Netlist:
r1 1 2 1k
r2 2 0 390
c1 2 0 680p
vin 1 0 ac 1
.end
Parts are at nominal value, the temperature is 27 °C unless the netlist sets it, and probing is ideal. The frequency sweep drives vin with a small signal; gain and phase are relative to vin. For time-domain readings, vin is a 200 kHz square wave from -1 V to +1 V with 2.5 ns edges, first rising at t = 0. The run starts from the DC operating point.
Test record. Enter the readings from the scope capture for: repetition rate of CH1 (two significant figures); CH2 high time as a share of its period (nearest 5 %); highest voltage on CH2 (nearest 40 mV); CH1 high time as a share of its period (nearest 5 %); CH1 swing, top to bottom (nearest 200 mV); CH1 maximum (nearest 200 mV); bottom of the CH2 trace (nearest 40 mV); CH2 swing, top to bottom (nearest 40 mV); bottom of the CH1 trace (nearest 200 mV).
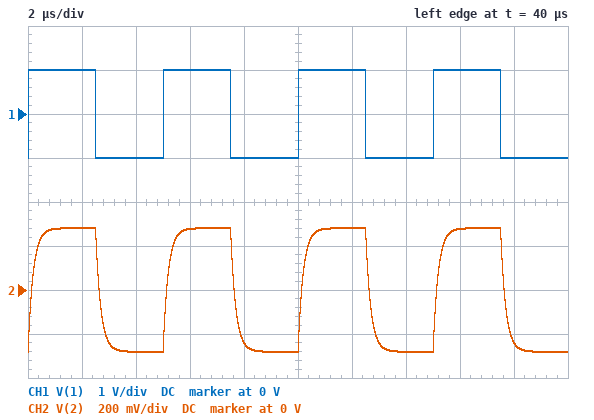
200 kHz
50 %
280 mV
50 %
2.0 V
1.0 V
-280 mV
560 mV
-1.0 V
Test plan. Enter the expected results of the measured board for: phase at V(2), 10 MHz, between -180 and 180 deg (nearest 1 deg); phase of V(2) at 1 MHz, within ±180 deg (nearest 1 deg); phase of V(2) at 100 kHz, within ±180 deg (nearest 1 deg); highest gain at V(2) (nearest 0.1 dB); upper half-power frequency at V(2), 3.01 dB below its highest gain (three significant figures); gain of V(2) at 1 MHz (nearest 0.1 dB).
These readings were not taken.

-85 deg
-50 deg
-7 deg
-11.0 dB
834 kHz
-14.9 dB
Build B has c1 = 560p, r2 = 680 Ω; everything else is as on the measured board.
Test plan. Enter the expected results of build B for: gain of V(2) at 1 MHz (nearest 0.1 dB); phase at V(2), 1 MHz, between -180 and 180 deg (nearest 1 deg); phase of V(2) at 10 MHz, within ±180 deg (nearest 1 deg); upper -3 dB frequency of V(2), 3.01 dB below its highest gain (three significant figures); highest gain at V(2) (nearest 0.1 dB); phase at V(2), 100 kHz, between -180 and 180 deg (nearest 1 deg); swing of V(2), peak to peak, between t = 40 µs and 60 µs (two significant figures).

-12.7 dB
-55 deg
-86 deg
702 kHz
-7.9 dB
-8 deg
810 mV
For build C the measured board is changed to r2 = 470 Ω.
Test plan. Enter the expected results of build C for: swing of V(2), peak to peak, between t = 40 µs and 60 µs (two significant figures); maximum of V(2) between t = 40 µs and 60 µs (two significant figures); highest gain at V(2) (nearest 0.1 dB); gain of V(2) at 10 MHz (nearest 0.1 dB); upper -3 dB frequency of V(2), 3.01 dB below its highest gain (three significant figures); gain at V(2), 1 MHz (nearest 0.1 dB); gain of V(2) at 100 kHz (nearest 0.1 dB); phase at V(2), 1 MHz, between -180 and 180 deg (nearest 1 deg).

640 mV
320 mV
-9.9 dB
-32.6 dB
732 kHz
-14.5 dB
-10.0 dB
-54 deg
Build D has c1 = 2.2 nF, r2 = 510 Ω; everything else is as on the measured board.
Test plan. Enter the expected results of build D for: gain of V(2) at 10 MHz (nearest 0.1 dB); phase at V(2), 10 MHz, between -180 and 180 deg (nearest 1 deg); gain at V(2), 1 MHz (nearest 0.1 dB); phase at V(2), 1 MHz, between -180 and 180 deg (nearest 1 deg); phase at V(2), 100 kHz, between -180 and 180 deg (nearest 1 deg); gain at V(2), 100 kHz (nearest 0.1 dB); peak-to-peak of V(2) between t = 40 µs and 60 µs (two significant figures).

-42.8 dB
-89 deg
-23.0 dB
-78 deg
-25 deg
-10.3 dB
630 mV
